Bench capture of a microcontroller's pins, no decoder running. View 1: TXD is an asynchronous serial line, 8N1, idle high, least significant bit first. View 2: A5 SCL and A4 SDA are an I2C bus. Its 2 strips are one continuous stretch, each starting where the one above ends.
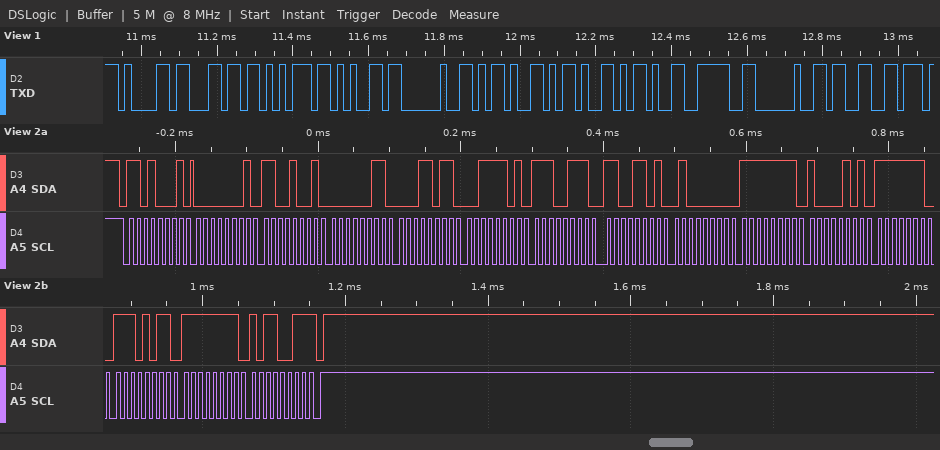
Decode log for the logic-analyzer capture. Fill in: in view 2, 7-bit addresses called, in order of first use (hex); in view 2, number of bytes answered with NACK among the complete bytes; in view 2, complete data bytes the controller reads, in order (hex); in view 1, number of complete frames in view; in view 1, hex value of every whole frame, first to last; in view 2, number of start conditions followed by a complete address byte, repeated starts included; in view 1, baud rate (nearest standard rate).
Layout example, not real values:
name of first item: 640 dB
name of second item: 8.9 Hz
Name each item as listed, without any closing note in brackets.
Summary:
in view 2, 7-bit addresses called, in order of first use: 0x68
in view 2, number of bytes answered with NACK among the complete bytes: 1
in view 2, complete data bytes the controller reads, in order: 01 C9 03 1B 3D E7 CD 40 FF 85 FE EB FF B3
in view 1, number of complete frames in view: 11
in view 1, hex value of every whole frame, first to last: 61 6C 75 65 20 2D 2D 2D 3E 20 33
in view 2, number of start conditions followed by a complete address byte, repeated starts included: 1
in view 1, baud rate: 57600 baud
